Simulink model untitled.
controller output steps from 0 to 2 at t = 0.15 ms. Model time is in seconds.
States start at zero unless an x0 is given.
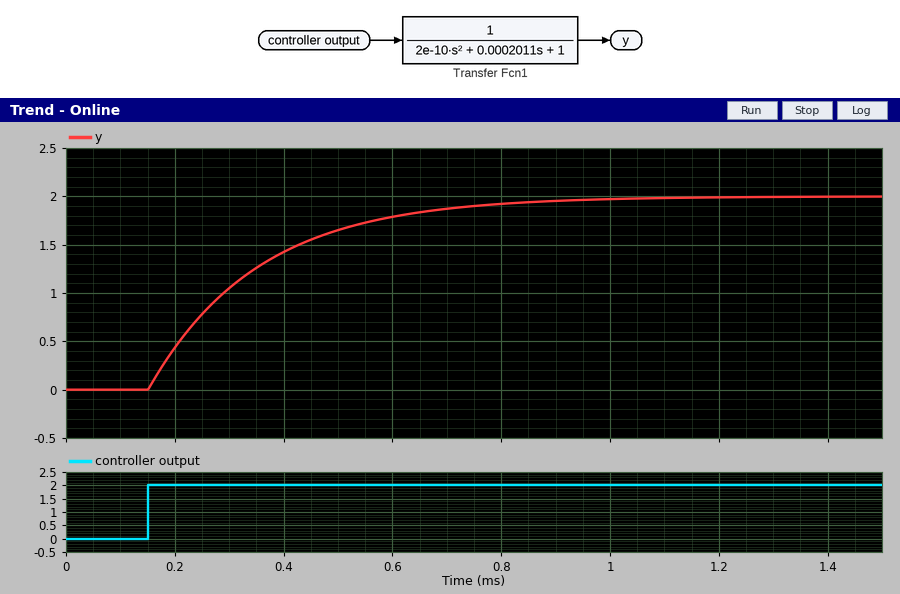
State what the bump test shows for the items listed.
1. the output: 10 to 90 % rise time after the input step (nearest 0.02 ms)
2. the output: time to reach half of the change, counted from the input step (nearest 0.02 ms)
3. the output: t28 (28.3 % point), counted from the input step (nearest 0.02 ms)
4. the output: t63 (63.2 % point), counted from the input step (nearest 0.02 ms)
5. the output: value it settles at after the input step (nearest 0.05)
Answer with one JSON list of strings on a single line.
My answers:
["0.44 ms", "0.14 ms", "0.06 ms", "0.20 ms", "2.00"]
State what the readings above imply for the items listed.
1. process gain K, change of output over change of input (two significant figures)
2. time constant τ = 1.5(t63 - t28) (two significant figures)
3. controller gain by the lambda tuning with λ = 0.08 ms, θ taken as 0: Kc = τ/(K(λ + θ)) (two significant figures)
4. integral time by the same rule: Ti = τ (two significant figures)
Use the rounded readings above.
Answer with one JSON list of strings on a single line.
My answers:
["1.0", "0.21 ms", "2.6", "0.21 ms"]
